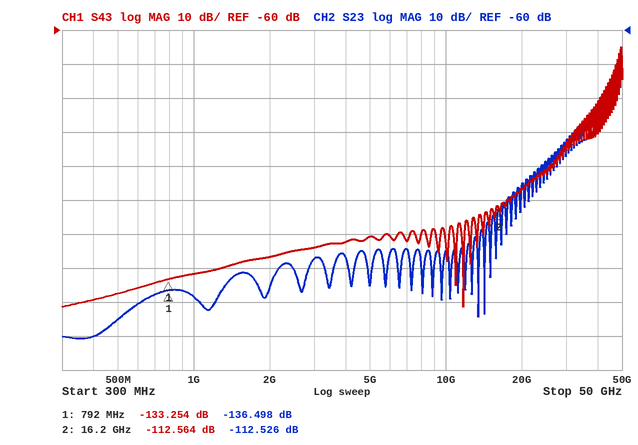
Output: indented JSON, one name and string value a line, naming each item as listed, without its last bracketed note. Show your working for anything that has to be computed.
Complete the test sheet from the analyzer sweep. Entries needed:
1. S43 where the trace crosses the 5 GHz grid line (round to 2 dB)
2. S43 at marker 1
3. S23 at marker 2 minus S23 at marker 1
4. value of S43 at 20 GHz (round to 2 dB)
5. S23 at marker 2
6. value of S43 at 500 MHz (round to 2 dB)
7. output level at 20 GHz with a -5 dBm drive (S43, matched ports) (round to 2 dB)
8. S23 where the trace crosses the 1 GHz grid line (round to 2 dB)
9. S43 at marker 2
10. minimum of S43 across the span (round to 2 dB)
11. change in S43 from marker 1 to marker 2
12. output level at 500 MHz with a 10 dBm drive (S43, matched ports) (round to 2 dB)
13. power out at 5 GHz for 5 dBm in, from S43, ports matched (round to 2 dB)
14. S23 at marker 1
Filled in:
{
  "S43 where the trace crosses the 5 GHz grid line": "-120 dB",
  "S43 at marker 1": "-133.254 dB",
  "S23 at marker 2 minus S23 at marker 1": "-112.526 − (-136.498) = 23.972 dB",
  "value of S43 at 20 GHz": "-106 dB",
  "S23 at marker 2": "-112.526 dB",
  "value of S43 at 500 MHz": "-138 dB",
  "output level at 20 GHz with a -5 dBm drive (S43, matched ports)": "-5 dBm + (-106 dB) = -112 dBm",
  "S23 where the trace crosses the 1 GHz grid line": "-138 dB",
  "S43 at marker 2": "-112.564 dB",
  "minimum of S43 across the span": "-142 dB",
  "change in S43 from marker 1 to marker 2": "-112.564 − (-133.254) = 20.690 dB",
  "output level at 500 MHz with a 10 dBm drive (S43, matched ports)": "10 dBm + (-138 dB) = -128 dBm",
  "power out at 5 GHz for 5 dBm in, from S43, ports matched": "5 dBm + (-120 dB) = -116 dBm",
  "S23 at marker 1": "-136.498 dB"
}
